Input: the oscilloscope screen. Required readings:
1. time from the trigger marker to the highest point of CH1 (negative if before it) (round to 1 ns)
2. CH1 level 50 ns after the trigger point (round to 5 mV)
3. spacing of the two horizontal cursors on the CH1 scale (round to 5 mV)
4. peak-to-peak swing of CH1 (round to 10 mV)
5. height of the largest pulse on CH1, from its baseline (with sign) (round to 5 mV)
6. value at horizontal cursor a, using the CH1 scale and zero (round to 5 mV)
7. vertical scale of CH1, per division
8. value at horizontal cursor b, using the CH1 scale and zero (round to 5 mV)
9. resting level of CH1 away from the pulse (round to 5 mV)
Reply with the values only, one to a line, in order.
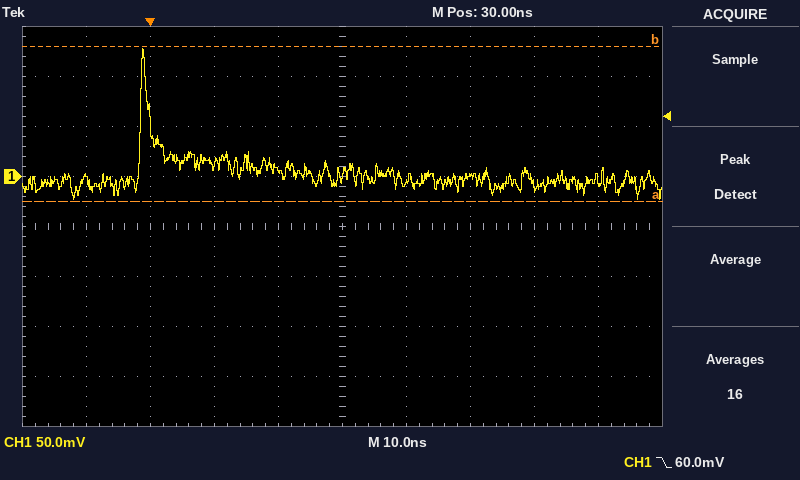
-1 ns
0 mV
155 mV
150 mV
+130 mV
-25 mV
50 mV
130 mV
-5 mV
